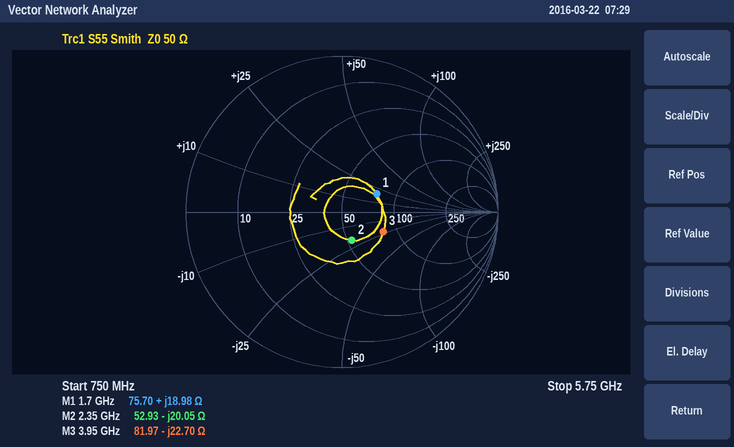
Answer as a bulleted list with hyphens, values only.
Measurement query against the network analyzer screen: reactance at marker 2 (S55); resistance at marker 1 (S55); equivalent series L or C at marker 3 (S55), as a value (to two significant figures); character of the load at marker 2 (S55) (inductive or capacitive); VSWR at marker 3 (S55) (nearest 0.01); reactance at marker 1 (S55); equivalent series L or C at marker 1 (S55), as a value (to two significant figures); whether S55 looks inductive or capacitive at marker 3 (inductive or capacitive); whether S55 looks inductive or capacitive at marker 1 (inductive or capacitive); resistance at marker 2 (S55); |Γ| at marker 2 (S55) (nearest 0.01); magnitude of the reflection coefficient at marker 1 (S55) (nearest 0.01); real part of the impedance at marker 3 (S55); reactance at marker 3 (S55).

- -20.05 Ω
- 75.70 Ω
- 1.8 pF
- capacitive
- 1.83
- +18.98 Ω
- 1.8 nH
- capacitive
- inductive
- 52.93 Ω
- 0.19
- 0.25
- 81.97 Ω
- -22.70 Ω
